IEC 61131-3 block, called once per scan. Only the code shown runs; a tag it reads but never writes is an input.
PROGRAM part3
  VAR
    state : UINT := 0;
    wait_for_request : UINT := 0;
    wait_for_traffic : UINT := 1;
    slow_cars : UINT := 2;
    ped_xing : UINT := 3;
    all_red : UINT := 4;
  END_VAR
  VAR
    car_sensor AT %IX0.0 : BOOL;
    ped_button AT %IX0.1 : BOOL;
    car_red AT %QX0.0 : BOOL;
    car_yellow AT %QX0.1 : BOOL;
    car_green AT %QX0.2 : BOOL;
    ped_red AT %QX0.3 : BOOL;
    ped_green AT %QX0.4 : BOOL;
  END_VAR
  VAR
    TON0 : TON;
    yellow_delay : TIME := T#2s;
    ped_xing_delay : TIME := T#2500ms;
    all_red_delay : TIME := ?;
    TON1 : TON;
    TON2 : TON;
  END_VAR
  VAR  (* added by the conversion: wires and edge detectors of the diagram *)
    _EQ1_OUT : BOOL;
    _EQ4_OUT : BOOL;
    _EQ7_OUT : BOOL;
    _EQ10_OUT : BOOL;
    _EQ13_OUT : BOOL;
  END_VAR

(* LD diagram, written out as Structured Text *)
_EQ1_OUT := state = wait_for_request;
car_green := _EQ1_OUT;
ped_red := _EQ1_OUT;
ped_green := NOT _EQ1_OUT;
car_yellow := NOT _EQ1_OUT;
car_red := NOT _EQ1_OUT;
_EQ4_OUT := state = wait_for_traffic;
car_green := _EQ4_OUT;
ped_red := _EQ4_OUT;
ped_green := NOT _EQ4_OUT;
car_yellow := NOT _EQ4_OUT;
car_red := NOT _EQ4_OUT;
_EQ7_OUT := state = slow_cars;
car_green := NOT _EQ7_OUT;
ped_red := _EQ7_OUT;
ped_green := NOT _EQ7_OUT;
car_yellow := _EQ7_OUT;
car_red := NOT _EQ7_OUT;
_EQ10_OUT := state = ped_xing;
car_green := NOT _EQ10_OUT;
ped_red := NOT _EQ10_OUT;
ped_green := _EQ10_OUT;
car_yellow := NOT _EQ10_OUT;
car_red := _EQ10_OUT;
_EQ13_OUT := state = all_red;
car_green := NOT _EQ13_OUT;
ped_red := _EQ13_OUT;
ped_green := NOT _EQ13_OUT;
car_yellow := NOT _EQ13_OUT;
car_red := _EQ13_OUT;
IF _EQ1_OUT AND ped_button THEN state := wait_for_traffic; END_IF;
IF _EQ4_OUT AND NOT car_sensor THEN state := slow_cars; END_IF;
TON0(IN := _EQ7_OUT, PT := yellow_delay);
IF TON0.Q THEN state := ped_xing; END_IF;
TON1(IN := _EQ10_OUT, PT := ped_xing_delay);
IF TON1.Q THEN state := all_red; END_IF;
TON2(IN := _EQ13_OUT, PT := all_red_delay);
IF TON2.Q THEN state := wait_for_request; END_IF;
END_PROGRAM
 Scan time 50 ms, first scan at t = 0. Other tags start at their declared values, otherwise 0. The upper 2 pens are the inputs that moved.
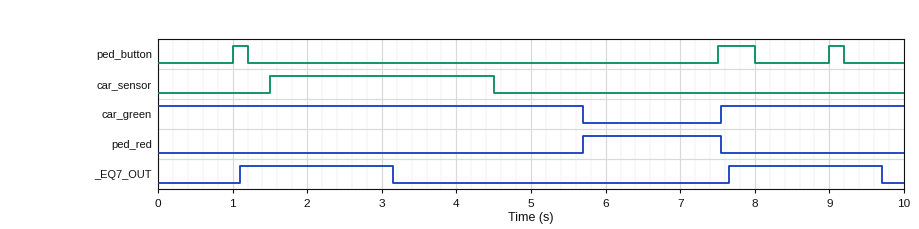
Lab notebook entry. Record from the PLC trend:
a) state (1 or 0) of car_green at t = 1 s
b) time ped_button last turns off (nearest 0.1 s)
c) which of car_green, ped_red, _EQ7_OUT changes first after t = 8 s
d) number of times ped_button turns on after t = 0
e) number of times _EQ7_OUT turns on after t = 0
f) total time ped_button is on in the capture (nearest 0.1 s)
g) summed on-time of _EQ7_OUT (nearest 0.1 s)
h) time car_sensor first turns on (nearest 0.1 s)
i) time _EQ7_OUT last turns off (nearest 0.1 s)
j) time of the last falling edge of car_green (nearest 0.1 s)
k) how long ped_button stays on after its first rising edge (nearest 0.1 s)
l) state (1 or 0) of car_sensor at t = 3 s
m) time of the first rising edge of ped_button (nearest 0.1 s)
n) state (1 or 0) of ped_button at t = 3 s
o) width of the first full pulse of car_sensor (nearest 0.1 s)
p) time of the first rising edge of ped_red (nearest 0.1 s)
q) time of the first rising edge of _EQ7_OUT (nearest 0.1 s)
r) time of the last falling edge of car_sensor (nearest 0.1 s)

1
9.2 s
_EQ7_OUT
3
2
0.9 s
4.1 s
1.5 s
9.7 s
5.7 s
0.2 s
1
1.0 s
0
3.0 s
5.7 s
1.1 s
4.5 s
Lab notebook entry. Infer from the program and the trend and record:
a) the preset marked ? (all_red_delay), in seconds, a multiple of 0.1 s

1.8 s
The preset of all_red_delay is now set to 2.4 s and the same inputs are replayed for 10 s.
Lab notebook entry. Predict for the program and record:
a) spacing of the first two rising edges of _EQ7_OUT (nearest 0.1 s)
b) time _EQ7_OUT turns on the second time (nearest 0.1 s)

8.0 s
9.1 s
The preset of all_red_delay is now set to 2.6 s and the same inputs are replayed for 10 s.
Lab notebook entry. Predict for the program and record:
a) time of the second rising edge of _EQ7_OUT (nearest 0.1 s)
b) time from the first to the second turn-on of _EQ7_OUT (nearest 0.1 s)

9.1 s
8.0 s
